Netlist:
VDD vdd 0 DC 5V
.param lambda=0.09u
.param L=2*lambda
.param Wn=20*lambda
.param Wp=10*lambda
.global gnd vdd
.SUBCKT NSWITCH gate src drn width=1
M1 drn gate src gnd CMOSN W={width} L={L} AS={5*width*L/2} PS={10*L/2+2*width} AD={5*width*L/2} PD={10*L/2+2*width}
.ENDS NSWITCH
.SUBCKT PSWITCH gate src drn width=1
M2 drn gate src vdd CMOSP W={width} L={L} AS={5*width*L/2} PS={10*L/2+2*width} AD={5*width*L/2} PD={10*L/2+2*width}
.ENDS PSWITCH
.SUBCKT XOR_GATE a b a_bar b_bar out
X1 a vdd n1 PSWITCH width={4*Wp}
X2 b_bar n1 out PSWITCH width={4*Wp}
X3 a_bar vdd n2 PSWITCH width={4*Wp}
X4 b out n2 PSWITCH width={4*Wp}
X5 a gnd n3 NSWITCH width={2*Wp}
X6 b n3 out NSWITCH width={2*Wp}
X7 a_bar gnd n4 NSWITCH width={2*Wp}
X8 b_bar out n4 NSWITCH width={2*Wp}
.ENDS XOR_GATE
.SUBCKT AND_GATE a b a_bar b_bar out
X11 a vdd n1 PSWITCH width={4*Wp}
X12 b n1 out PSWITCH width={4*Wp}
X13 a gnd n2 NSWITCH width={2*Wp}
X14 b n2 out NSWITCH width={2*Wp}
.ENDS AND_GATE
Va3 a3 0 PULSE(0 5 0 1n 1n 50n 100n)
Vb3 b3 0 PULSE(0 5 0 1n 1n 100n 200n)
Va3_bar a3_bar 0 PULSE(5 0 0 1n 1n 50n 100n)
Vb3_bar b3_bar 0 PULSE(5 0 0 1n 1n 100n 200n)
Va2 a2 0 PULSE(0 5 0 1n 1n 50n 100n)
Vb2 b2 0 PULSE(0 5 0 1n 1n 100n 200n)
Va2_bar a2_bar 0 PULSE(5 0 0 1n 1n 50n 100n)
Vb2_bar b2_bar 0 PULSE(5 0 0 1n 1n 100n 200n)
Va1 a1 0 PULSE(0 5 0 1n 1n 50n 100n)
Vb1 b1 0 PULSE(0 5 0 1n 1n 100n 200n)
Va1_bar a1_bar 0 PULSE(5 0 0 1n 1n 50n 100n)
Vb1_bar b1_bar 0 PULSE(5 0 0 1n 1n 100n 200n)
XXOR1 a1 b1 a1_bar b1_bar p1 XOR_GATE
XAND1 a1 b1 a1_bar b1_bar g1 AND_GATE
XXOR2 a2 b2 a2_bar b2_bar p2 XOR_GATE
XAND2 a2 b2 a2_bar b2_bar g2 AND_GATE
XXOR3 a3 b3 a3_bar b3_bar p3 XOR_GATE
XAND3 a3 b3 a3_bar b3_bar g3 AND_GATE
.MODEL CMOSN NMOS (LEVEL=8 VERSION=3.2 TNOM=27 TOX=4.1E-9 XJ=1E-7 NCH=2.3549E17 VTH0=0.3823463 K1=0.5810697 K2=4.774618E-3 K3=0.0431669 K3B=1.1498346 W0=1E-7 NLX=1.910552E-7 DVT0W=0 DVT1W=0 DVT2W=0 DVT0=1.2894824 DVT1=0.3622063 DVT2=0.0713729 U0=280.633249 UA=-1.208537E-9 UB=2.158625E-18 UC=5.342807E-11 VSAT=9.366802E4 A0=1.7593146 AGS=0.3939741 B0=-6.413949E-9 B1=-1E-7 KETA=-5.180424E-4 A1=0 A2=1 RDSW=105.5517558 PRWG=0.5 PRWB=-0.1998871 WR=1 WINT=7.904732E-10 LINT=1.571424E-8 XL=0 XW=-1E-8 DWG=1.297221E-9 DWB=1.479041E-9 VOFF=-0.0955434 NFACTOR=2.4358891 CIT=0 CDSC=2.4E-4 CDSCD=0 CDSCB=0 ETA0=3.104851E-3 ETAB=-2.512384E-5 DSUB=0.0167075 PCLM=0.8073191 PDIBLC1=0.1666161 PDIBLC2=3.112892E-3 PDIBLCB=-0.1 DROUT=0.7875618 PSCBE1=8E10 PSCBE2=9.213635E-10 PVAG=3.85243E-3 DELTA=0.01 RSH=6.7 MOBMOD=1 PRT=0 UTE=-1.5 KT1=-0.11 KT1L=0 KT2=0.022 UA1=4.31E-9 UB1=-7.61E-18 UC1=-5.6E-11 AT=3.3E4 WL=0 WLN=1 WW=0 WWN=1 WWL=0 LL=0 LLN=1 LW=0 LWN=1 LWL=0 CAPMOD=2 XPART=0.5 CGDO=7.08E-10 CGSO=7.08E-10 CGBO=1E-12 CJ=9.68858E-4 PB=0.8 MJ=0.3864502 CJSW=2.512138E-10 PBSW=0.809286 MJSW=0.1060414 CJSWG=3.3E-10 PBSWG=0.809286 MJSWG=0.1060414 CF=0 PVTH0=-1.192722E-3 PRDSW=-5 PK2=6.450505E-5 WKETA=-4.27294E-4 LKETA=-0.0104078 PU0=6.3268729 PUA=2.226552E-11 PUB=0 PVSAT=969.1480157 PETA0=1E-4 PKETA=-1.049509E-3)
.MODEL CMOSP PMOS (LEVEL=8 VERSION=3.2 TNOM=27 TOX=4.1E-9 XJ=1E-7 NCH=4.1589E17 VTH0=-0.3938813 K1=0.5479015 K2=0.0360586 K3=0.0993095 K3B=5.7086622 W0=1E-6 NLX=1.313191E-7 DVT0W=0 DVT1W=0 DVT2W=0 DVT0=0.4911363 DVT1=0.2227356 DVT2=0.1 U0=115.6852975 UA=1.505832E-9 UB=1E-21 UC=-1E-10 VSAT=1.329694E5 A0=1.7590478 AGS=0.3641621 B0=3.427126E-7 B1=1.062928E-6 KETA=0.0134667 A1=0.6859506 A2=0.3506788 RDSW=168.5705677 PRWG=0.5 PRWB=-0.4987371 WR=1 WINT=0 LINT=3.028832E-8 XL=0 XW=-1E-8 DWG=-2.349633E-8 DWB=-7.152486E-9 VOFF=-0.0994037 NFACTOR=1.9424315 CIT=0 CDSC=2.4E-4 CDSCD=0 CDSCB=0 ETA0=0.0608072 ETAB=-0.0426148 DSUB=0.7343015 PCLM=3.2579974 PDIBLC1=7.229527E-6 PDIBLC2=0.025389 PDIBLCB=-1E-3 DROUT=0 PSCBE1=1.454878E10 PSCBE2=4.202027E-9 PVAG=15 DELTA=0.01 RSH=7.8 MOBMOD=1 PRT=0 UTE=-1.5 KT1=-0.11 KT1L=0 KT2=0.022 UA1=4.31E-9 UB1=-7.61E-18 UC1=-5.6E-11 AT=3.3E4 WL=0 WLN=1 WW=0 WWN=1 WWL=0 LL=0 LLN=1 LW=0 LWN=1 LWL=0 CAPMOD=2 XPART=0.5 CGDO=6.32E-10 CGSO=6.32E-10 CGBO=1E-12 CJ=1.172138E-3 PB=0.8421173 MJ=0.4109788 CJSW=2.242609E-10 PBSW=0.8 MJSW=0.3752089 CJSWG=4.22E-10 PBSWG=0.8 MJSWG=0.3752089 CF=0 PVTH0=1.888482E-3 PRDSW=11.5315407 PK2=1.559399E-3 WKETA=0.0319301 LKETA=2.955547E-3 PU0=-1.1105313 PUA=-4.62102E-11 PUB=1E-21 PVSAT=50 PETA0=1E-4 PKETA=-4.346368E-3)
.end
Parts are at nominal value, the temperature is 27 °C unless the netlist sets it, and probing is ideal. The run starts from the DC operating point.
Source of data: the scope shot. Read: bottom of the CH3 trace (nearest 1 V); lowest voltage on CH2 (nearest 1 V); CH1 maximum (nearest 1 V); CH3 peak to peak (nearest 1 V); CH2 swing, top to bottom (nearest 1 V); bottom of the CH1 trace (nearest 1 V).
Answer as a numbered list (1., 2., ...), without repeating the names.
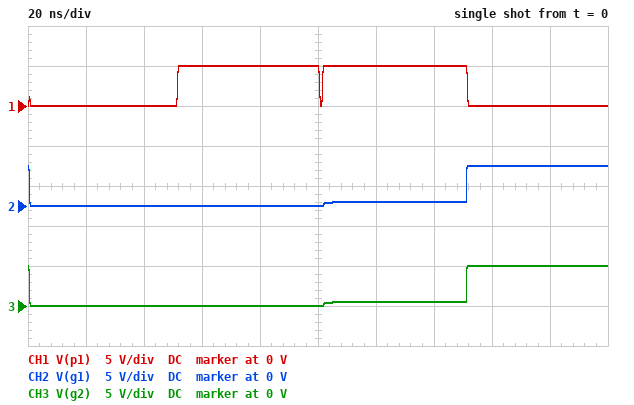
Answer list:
1. 0 V
2. 0 V
3. 5 V
4. 5 V
5. 5 V
6. 0 V
